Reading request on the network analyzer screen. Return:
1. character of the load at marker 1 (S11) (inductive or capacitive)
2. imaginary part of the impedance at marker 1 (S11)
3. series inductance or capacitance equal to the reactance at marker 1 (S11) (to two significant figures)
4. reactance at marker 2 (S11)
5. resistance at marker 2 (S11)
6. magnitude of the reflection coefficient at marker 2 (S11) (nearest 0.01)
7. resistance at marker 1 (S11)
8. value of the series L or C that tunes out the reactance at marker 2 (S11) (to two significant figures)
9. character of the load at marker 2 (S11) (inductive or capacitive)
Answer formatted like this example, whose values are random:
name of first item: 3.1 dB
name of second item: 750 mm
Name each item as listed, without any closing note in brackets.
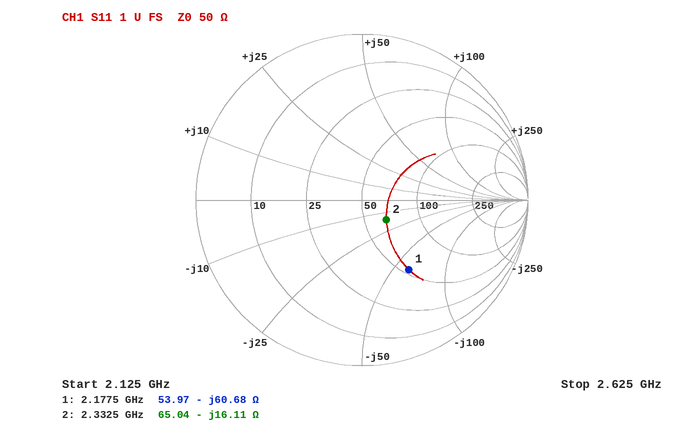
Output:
character of the load at marker 1 (S11): capacitive
imaginary part of the impedance at marker 1: -60.68 Ω
series inductance or capacitance equal to the reactance at marker 1 (S11): 1.2 pF
reactance at marker 2: -16.11 Ω
resistance at marker 2: 65.04 Ω
magnitude of the reflection coefficient at marker 2 (S11): 0.19
resistance at marker 1: 53.97 Ω
value of the series L or C that tunes out the reactance at marker 2 (S11): 1.1 nH
character of the load at marker 2 (S11): capacitive
